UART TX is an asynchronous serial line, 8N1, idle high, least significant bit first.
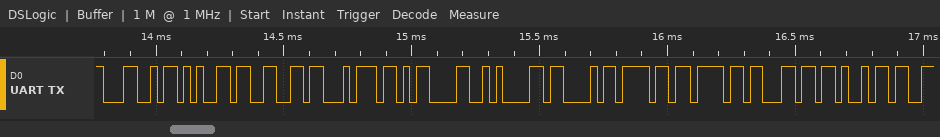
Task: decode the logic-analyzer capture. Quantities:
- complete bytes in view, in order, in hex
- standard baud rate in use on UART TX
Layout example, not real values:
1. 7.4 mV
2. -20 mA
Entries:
1. 0x4C 0x65 0x66 0x74 0x0D 0x0A 0x43 0x6F 0x6F 0x6C 0x69
2. 38400 baud
